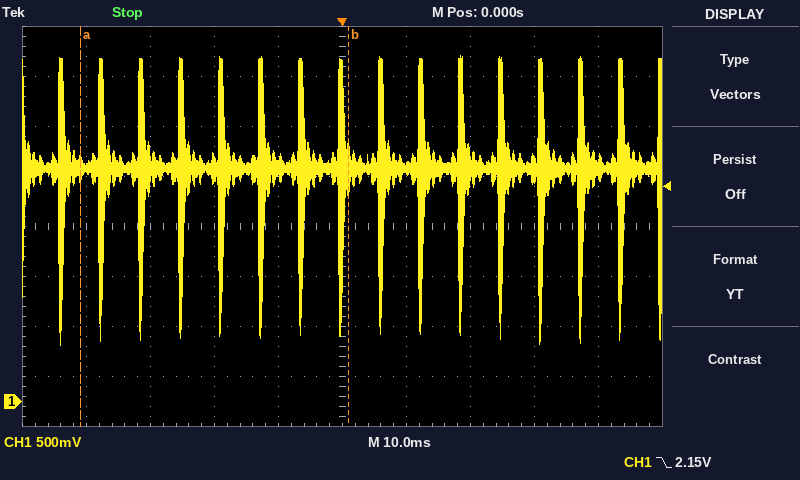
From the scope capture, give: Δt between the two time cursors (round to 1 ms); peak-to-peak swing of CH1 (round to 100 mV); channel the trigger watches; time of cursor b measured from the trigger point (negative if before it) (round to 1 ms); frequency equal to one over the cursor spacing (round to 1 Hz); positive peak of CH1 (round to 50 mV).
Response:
42 ms
2.90 V
CH1
+1 ms
24 Hz
3.45 V
